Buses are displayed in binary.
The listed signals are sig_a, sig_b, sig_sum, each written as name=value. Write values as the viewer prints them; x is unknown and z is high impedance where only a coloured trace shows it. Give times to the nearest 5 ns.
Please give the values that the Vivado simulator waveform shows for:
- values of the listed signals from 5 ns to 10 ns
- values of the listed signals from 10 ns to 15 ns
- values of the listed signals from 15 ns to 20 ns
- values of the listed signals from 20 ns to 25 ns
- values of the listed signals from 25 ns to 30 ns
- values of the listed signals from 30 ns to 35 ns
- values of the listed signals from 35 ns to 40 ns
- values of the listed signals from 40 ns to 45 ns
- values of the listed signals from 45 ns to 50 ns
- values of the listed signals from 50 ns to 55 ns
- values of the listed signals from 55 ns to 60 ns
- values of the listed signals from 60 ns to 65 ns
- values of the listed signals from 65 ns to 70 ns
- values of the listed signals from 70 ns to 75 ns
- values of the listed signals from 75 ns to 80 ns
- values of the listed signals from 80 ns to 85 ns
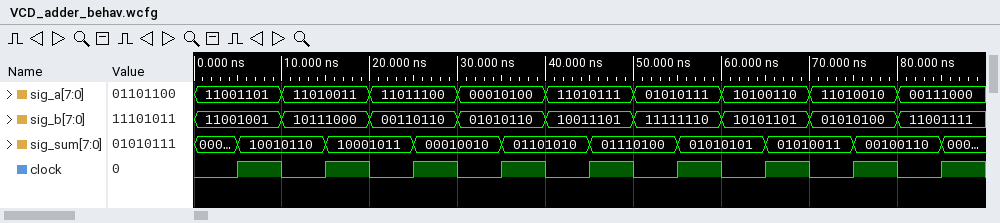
sig_a=11001101, sig_b=11001001, sig_sum=10010110
sig_a=11010011, sig_b=10111000, sig_sum=10010110
sig_a=11010011, sig_b=10111000, sig_sum=10001011
sig_a=11011100, sig_b=00110110, sig_sum=10001011
sig_a=11011100, sig_b=00110110, sig_sum=00010010
sig_a=00010100, sig_b=01010110, sig_sum=00010010
sig_a=00010100, sig_b=01010110, sig_sum=01101010
sig_a=11010111, sig_b=10011101, sig_sum=01101010
sig_a=11010111, sig_b=10011101, sig_sum=01110100
sig_a=01010111, sig_b=11111110, sig_sum=01110100
sig_a=01010111, sig_b=11111110, sig_sum=01010101
sig_a=10100110, sig_b=10101101, sig_sum=01010101
sig_a=10100110, sig_b=10101101, sig_sum=01010011
sig_a=11010010, sig_b=01010100, sig_sum=01010011
sig_a=11010010, sig_b=01010100, sig_sum=00100110
sig_a=00111000, sig_b=11001111, sig_sum=00100110
